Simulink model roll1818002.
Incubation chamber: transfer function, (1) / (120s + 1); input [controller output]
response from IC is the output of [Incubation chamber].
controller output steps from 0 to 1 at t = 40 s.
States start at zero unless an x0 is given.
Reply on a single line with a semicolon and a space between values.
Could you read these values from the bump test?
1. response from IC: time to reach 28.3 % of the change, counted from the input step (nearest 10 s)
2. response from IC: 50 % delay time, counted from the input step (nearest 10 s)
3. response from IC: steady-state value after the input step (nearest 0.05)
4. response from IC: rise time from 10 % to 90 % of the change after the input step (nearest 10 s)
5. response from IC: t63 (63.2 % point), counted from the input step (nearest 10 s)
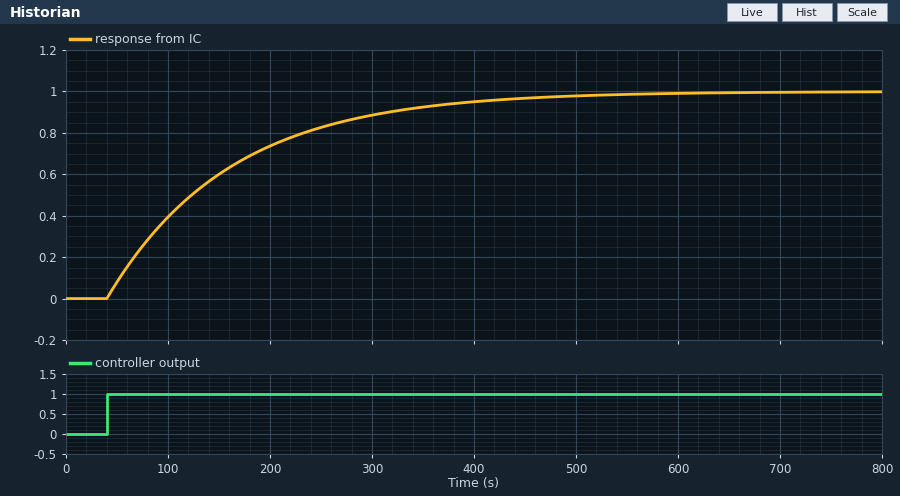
40 s; 80 s; 1.00; 260 s; 120 s
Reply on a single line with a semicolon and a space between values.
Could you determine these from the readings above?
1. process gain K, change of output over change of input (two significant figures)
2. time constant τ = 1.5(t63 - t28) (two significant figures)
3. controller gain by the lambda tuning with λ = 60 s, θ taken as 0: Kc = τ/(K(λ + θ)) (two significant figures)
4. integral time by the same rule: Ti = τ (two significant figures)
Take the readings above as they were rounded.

1.0; 120 s; 2.0; 120 s
